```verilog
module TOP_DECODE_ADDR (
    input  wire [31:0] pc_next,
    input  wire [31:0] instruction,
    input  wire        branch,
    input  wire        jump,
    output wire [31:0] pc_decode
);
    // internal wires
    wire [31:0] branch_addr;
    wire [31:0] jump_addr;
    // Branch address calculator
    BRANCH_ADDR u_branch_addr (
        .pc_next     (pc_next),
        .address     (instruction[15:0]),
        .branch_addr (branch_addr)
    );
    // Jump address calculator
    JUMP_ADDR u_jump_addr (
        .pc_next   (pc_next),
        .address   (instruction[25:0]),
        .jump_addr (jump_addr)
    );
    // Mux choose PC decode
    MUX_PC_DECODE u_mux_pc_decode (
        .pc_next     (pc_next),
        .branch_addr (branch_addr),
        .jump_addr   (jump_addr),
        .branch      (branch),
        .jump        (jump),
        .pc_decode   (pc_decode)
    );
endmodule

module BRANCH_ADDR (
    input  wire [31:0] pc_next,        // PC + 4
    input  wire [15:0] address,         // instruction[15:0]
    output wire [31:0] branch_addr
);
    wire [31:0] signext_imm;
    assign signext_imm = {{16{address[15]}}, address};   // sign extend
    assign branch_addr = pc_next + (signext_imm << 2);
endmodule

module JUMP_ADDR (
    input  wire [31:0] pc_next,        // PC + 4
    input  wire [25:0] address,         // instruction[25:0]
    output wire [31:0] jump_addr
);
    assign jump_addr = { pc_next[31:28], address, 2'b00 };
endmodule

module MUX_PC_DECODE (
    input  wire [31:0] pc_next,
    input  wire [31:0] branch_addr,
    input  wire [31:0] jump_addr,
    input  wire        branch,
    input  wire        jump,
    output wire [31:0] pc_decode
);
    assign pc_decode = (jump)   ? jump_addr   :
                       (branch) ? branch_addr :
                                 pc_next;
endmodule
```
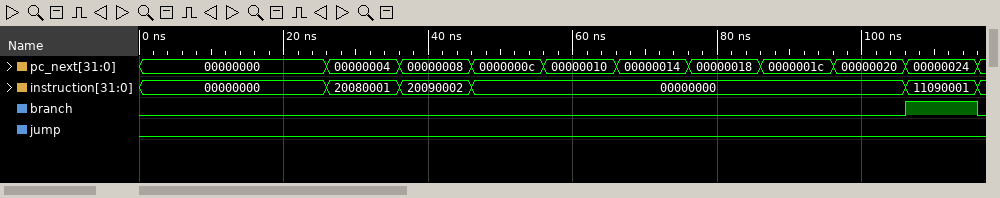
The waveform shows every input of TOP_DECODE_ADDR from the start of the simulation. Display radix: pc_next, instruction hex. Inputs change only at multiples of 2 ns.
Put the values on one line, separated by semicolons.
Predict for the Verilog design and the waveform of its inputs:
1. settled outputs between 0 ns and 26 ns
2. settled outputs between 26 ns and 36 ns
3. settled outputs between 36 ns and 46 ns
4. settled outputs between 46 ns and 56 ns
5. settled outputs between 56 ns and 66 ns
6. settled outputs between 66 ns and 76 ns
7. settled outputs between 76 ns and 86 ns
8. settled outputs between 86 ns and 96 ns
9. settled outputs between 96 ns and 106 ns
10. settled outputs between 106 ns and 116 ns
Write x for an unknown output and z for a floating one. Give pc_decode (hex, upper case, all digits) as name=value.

pc_decode=00000000; pc_decode=00000004; pc_decode=00000008; pc_decode=0000000C; pc_decode=00000010; pc_decode=00000014; pc_decode=00000018; pc_decode=0000001C; pc_decode=00000020; pc_decode=00000028
